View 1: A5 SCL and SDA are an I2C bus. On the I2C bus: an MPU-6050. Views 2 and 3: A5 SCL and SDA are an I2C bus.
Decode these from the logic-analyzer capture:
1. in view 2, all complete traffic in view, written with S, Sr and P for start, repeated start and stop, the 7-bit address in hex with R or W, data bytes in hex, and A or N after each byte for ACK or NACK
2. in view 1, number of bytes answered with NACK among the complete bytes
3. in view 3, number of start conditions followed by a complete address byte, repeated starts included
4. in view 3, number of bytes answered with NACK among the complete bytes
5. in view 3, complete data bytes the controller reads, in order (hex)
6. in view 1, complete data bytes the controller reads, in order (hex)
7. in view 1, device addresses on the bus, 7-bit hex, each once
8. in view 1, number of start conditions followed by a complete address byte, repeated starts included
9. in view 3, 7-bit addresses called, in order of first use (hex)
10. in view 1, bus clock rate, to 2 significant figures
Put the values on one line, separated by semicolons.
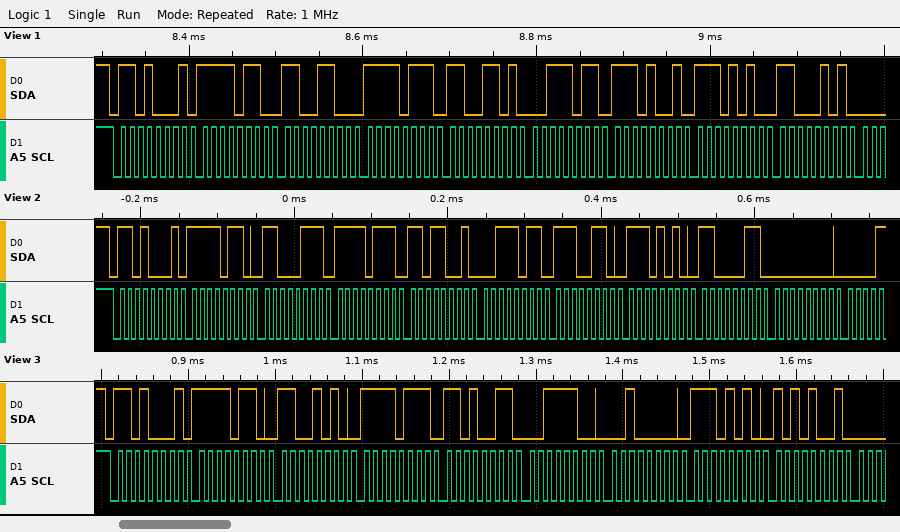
S 68R A F6 A C7 A F7 A D9 A 3B A E6 A EA A C3 A 00 A; 0; 1; 0; F6 CA F7 D3 3C 20 EA A9; F6 CC F7 CD 3B E9 EA C5; 0x68; 1; 0x68; 100 kHz
